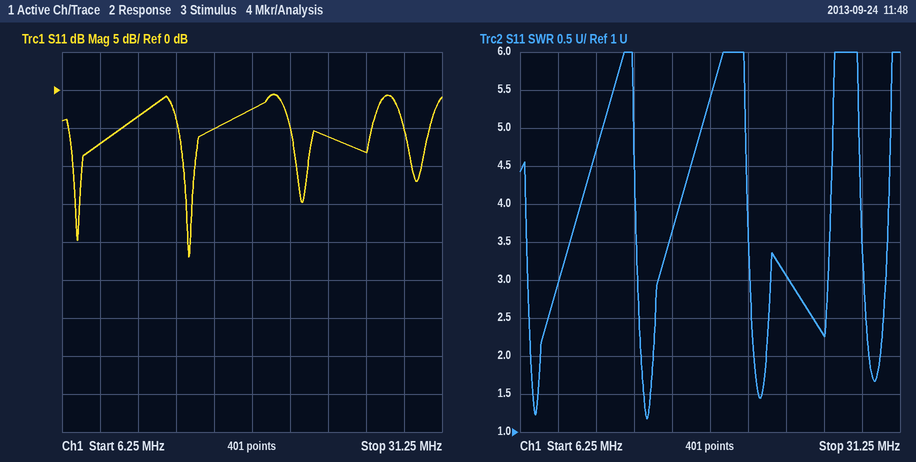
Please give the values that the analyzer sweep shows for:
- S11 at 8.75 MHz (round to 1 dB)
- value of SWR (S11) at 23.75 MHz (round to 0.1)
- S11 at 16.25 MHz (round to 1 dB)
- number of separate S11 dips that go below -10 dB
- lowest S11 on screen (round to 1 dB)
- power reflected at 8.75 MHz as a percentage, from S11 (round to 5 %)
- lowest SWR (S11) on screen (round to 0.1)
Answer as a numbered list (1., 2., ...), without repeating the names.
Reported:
1. -7 dB
2. 3.1
3. -5 dB
4. 4
5. -22 dB
6. 20 %
7. 1.2
